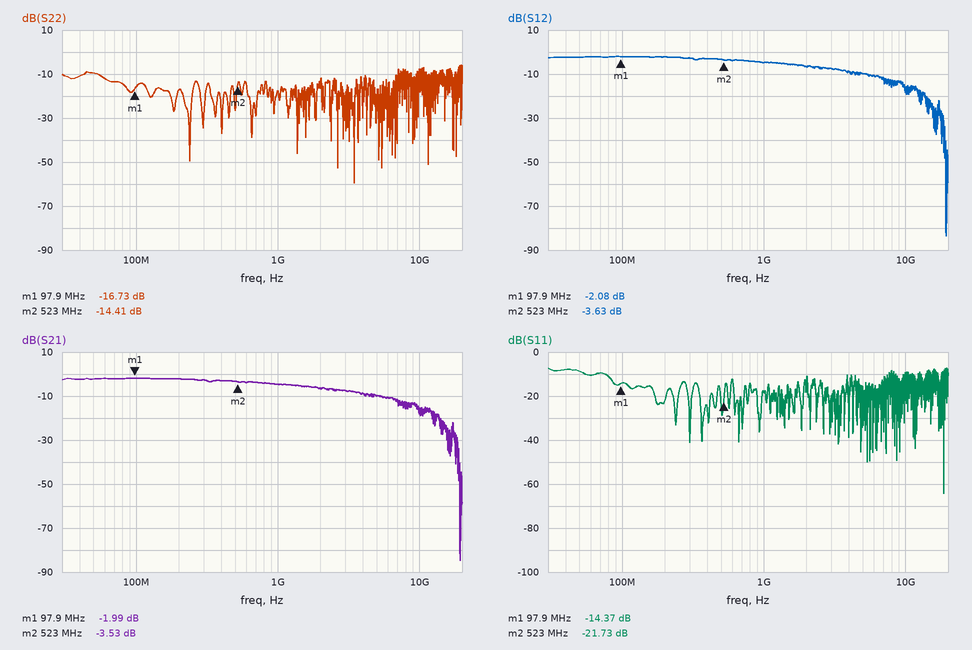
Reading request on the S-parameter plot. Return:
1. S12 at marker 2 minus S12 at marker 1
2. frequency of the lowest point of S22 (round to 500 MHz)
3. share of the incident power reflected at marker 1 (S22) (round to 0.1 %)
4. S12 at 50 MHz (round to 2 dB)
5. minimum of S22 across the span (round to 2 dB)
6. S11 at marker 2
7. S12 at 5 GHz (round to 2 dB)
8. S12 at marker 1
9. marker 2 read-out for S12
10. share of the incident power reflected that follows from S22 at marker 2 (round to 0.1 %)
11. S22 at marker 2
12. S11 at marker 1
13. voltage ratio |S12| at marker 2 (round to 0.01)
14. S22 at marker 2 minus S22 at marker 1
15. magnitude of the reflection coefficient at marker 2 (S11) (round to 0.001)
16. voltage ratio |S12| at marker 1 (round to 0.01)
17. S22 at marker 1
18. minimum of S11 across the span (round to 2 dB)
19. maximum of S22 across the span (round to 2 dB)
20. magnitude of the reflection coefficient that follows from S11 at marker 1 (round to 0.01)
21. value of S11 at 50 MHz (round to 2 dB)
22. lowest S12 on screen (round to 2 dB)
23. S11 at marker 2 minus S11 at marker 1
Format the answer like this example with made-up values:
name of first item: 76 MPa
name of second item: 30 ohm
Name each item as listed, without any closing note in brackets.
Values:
S12 at marker 2 minus S12 at marker 1: -1.55 dB
frequency of the lowest point of S22: 3.5 GHz
share of the incident power reflected at marker 1 (S22): 2.1 %
S12 at 50 MHz: -2 dB
minimum of S22 across the span: -60 dB
S11 at marker 2: -21.73 dB
S12 at 5 GHz: -10 dB
S12 at marker 1: -2.08 dB
marker 2 read-out for S12: -3.63 dB
share of the incident power reflected that follows from S22 at marker 2: 3.6 %
S22 at marker 2: -14.41 dB
S11 at marker 1: -14.37 dB
voltage ratio |S12| at marker 2: 0.66
S22 at marker 2 minus S22 at marker 1: 2.32 dB
magnitude of the reflection coefficient at marker 2 (S11): 0.082
voltage ratio |S12| at marker 1: 0.79
S22 at marker 1: -16.73 dB
minimum of S11 across the span: -64 dB
maximum of S22 across the span: -6 dB
magnitude of the reflection coefficient that follows from S11 at marker 1: 0.19
value of S11 at 50 MHz: -8 dB
lowest S12 on screen: -84 dB
S11 at marker 2 minus S11 at marker 1: -7.36 dB
